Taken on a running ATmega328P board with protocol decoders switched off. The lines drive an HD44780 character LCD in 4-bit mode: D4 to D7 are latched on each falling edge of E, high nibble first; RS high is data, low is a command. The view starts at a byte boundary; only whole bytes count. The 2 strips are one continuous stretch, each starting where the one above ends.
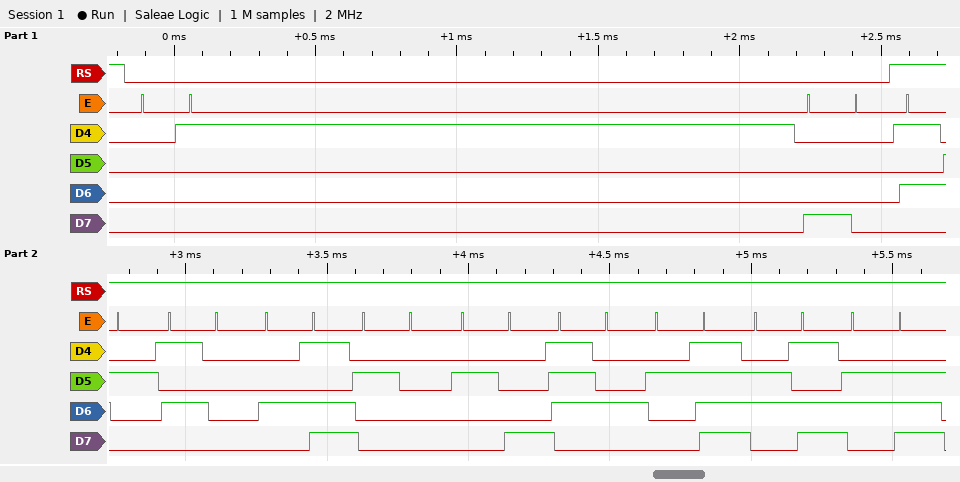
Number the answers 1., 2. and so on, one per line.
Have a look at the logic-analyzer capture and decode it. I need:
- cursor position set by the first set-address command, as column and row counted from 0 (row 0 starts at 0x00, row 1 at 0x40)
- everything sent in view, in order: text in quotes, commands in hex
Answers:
1. column 0, row 0
2. 0x01 0x80 "RPM (t/mn"
